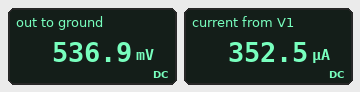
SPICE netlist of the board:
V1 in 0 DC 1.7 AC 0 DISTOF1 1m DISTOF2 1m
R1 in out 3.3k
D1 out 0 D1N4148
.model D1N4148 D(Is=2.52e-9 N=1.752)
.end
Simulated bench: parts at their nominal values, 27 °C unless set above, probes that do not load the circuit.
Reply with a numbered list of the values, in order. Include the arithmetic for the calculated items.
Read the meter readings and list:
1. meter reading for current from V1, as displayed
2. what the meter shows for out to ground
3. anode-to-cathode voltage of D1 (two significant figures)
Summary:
1. 352.5 µA
2. 536.9 mV
3. 536.9 mV = 540 mV
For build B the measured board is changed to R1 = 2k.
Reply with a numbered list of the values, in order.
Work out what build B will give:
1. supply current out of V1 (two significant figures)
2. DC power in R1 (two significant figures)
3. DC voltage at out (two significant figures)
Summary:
1. 570 µA
2. 650 µW
3. 560 mV
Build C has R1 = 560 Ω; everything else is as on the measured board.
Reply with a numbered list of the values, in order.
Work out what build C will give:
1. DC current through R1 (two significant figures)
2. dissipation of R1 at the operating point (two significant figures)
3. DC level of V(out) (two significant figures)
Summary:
1. 1.9 mA
2. 2.1 mW
3. 610 mV
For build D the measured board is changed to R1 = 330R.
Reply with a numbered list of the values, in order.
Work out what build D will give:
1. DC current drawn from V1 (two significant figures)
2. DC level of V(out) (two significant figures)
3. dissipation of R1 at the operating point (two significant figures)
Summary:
1. 3.2 mA
2. 640 mV
3. 3.4 mW
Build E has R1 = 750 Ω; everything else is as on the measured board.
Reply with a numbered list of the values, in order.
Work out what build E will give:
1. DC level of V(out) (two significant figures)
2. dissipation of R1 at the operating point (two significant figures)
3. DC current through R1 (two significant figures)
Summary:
1. 600 mV
2. 1.6 mW
3. 1.5 mA
